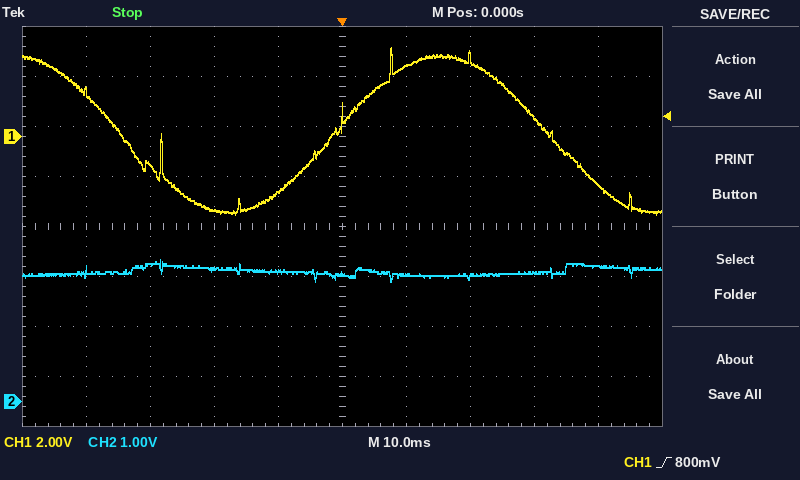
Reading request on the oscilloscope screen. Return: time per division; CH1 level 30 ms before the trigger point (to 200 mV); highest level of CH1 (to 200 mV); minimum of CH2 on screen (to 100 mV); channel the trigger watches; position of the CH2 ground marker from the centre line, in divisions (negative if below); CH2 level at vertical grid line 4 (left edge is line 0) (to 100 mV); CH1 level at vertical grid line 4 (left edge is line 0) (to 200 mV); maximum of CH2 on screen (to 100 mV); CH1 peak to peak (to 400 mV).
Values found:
10 ms
-1.2 V
3.6 V
2.4 V
CH1
-3.5 div
2.6 V
-2.2 V
2.8 V
6.8 V
